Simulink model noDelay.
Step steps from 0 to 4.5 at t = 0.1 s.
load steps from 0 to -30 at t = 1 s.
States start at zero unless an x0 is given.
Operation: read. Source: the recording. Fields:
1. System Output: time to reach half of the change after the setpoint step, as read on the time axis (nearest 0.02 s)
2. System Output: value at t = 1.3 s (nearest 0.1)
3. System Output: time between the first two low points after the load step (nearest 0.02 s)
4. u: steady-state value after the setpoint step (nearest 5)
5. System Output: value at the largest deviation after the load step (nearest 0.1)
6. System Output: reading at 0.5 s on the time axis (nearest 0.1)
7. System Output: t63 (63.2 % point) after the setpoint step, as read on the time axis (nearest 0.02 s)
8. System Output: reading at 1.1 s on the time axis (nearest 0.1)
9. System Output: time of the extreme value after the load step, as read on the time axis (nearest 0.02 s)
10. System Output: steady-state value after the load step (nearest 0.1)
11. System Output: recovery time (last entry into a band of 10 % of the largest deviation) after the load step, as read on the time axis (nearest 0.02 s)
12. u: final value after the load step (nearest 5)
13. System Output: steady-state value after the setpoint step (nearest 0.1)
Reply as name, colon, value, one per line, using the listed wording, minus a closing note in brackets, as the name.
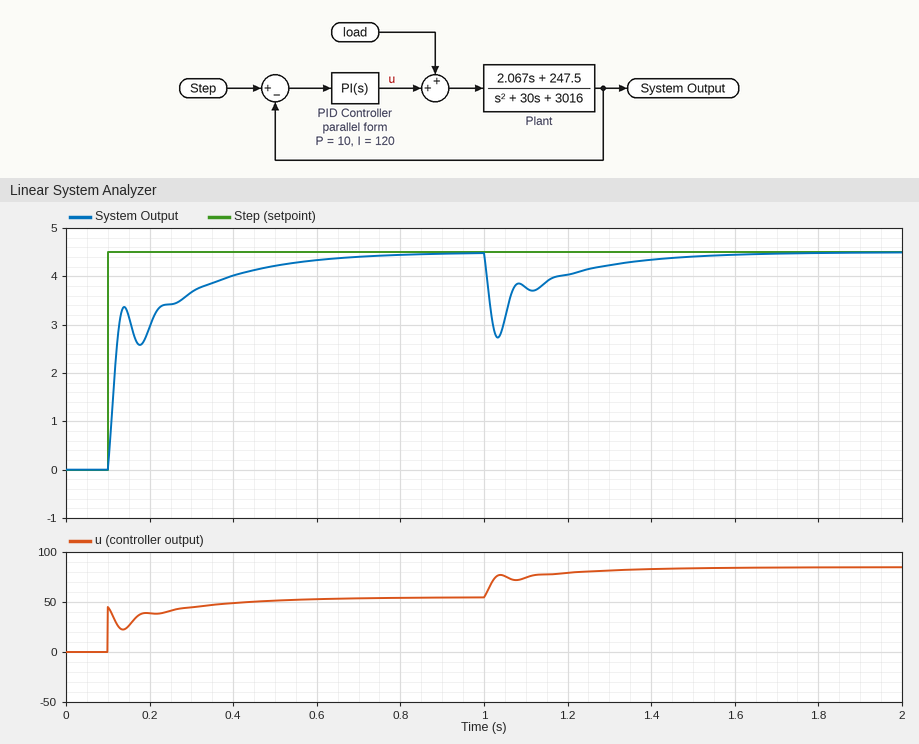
System Output: time to reach half of the change after the setpoint step, as read on the time axis: 0.12 s
System Output: value at t = 1.3 s: 4.2
System Output: time between the first two low points after the load step: 0.08 s
u: steady-state value after the setpoint step: 55
System Output: value at the largest deviation after the load step: 2.7
System Output: reading at 0.5 s on the time axis: 4.2
System Output: t63 (63.2 % point) after the setpoint step, as read on the time axis: 0.12 s
System Output: reading at 1.1 s on the time axis: 3.8
System Output: time of the extreme value after the load step, as read on the time axis: 1.04 s
System Output: steady-state value after the load step: 4.5
System Output: recovery time (last entry into a band of 10 % of the largest deviation) after the load step, as read on the time axis: 1.38 s
u: final value after the load step: 85
System Output: steady-state value after the setpoint step: 4.5
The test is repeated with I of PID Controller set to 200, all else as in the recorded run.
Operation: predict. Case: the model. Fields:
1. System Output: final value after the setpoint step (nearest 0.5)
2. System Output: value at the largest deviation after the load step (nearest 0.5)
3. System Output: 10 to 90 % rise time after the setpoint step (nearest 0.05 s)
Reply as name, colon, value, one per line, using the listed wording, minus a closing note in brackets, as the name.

System Output: final value after the setpoint step: 4.5
System Output: value at the largest deviation after the load step: 3.0
System Output: 10 to 90 % rise time after the setpoint step: 0.20 s
